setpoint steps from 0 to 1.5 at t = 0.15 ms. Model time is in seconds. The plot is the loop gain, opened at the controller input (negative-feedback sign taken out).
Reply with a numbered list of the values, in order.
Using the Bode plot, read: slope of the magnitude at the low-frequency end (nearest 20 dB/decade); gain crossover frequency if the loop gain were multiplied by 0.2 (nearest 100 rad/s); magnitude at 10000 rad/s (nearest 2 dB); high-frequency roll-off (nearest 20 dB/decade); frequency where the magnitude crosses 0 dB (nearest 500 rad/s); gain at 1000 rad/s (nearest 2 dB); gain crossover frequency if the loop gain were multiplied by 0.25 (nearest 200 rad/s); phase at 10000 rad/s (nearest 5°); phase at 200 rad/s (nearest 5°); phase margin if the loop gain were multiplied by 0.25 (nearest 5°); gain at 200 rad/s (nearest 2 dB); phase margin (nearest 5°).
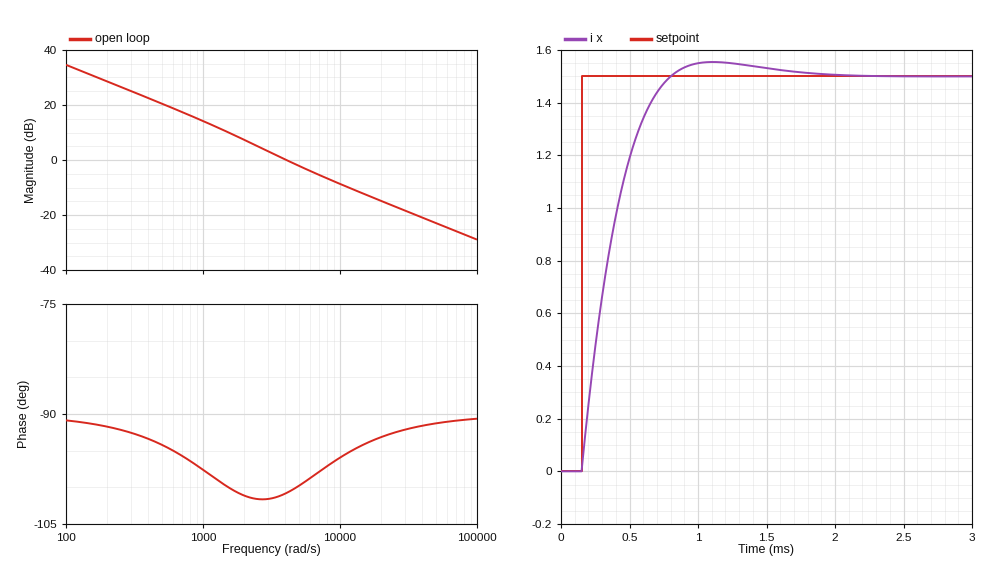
1. -20 dB/decade
2. 1000 rad/s
3. -8 dB
4. -20 dB/decade
5. 4000 rad/s
6. 14 dB
7. 1200 rad/s
8. -95°
9. -90°
10. 80°
11. 28 dB
12. 80°
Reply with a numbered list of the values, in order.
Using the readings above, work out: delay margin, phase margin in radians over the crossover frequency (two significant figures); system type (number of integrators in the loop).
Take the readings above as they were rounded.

1. 0.00035 s
2. 1
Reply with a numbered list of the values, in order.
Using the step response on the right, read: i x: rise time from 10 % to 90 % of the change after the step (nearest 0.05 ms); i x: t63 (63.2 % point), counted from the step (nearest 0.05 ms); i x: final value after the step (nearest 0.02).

1. 0.45 ms
2. 0.25 ms
3. 1.50
